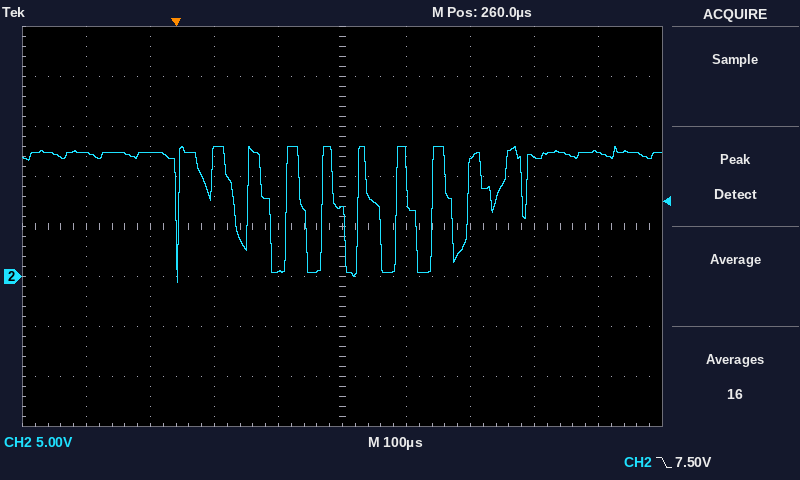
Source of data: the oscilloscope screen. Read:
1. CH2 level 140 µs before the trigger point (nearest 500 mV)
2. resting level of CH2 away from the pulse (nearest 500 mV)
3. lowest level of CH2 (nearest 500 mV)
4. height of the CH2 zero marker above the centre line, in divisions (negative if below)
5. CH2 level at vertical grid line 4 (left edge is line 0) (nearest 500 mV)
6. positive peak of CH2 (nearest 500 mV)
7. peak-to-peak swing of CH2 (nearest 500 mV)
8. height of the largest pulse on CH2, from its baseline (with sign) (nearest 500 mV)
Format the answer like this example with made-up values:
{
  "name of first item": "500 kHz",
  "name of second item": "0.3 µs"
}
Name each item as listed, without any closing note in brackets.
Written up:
{
  "CH2 level 140 µs before the trigger point": "12.5 V",
  "resting level of CH2 away from the pulse": "12.5 V",
  "lowest level of CH2": "-500 mV",
  "height of the CH2 zero marker above the centre line, in divisions": "-1.0 div",
  "CH2 level at vertical grid line 4 (left edge is line 0)": "500 mV",
  "positive peak of CH2": "13.0 V",
  "peak-to-peak swing of CH2": "13.5 V",
  "height of the largest pulse on CH2, from its baseline (with sign)": "-13.0 V"
}
